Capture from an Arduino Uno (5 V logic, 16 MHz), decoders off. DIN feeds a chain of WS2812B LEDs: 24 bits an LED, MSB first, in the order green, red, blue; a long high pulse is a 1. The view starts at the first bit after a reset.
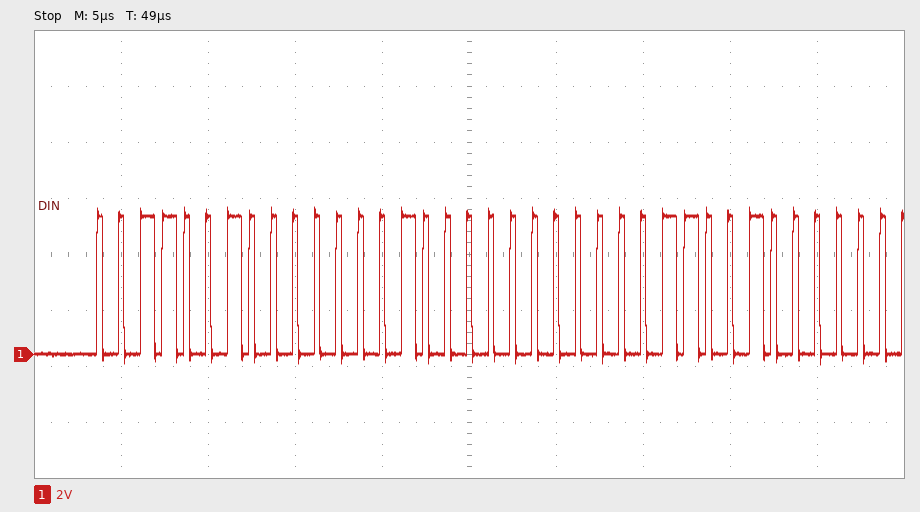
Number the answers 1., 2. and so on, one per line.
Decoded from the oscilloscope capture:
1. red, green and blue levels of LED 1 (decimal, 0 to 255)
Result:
1. 2, 50, 0
